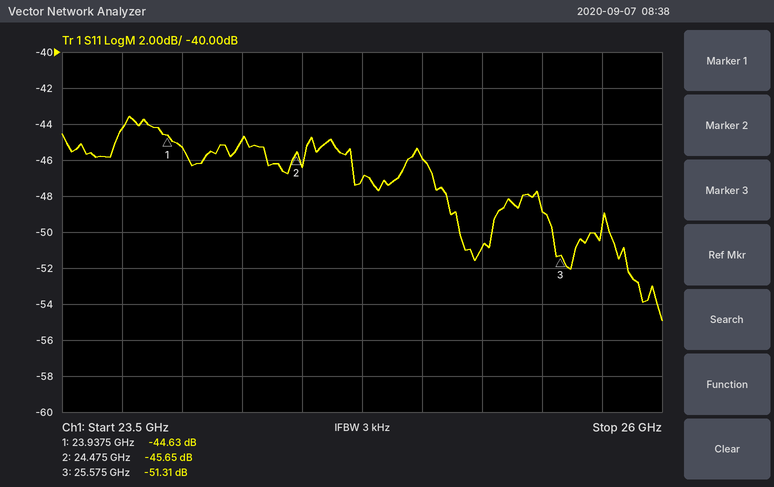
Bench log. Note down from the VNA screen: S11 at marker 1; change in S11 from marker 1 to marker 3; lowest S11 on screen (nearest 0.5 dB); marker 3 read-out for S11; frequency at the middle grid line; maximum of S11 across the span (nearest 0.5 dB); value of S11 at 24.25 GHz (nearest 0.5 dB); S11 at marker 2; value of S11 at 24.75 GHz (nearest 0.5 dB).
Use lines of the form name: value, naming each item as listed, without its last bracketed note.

S11 at marker 1: -44.63 dB
change in S11 from marker 1 to marker 3: -6.68 dB
lowest S11 on screen: -55.0 dB
marker 3 read-out for S11: -51.31 dB
frequency at the middle grid line: 24.75 GHz
maximum of S11 across the span: -43.5 dB
value of S11 at 24.25 GHz: -45.0 dB
S11 at marker 2: -45.65 dB
value of S11 at 24.75 GHz: -47.0 dB
